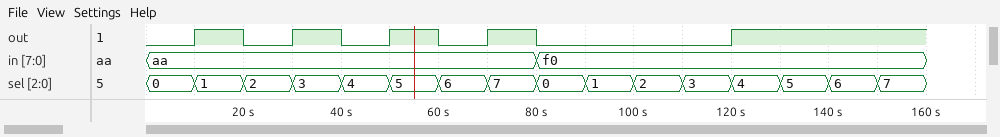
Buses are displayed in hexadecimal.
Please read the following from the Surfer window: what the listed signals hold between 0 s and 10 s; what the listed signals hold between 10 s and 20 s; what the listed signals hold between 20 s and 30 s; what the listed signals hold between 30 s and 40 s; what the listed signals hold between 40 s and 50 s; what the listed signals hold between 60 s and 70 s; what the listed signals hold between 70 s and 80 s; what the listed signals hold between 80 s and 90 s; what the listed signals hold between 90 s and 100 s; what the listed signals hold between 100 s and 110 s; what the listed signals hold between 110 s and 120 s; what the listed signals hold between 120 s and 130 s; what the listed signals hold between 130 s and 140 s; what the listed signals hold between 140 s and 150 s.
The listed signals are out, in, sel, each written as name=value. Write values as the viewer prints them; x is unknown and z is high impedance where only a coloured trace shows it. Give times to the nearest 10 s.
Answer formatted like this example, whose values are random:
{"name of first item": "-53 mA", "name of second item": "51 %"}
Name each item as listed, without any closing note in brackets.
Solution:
{"what the listed signals hold between 0 s and 10 s": "out=0, in=aa, sel=0", "what the listed signals hold between 10 s and 20 s": "out=1, in=aa, sel=1", "what the listed signals hold between 20 s and 30 s": "out=0, in=aa, sel=2", "what the listed signals hold between 30 s and 40 s": "out=1, in=aa, sel=3", "what the listed signals hold between 40 s and 50 s": "out=0, in=aa, sel=4", "what the listed signals hold between 60 s and 70 s": "out=0, in=aa, sel=6", "what the listed signals hold between 70 s and 80 s": "out=1, in=aa, sel=7", "what the listed signals hold between 80 s and 90 s": "out=0, in=f0, sel=0", "what the listed signals hold between 90 s and 100 s": "out=0, in=f0, sel=1", "what the listed signals hold between 100 s and 110 s": "out=0, in=f0, sel=2", "what the listed signals hold between 110 s and 120 s": "out=0, in=f0, sel=3", "what the listed signals hold between 120 s and 130 s": "out=1, in=f0, sel=4", "what the listed signals hold between 130 s and 140 s": "out=1, in=f0, sel=5", "what the listed signals hold between 140 s and 150 s": "out=1, in=f0, sel=6"}
